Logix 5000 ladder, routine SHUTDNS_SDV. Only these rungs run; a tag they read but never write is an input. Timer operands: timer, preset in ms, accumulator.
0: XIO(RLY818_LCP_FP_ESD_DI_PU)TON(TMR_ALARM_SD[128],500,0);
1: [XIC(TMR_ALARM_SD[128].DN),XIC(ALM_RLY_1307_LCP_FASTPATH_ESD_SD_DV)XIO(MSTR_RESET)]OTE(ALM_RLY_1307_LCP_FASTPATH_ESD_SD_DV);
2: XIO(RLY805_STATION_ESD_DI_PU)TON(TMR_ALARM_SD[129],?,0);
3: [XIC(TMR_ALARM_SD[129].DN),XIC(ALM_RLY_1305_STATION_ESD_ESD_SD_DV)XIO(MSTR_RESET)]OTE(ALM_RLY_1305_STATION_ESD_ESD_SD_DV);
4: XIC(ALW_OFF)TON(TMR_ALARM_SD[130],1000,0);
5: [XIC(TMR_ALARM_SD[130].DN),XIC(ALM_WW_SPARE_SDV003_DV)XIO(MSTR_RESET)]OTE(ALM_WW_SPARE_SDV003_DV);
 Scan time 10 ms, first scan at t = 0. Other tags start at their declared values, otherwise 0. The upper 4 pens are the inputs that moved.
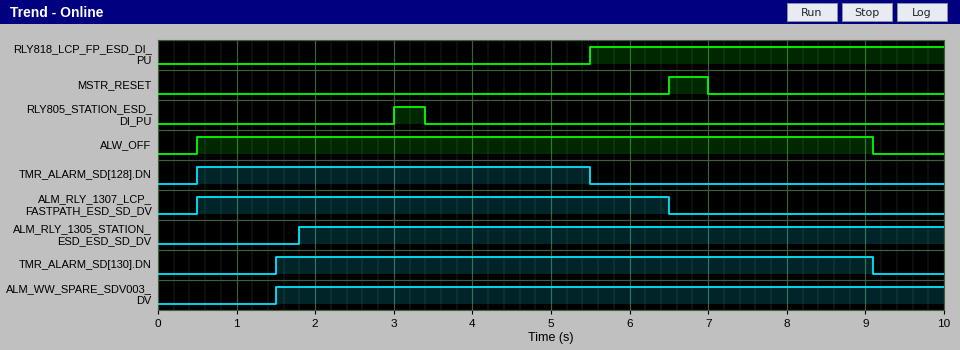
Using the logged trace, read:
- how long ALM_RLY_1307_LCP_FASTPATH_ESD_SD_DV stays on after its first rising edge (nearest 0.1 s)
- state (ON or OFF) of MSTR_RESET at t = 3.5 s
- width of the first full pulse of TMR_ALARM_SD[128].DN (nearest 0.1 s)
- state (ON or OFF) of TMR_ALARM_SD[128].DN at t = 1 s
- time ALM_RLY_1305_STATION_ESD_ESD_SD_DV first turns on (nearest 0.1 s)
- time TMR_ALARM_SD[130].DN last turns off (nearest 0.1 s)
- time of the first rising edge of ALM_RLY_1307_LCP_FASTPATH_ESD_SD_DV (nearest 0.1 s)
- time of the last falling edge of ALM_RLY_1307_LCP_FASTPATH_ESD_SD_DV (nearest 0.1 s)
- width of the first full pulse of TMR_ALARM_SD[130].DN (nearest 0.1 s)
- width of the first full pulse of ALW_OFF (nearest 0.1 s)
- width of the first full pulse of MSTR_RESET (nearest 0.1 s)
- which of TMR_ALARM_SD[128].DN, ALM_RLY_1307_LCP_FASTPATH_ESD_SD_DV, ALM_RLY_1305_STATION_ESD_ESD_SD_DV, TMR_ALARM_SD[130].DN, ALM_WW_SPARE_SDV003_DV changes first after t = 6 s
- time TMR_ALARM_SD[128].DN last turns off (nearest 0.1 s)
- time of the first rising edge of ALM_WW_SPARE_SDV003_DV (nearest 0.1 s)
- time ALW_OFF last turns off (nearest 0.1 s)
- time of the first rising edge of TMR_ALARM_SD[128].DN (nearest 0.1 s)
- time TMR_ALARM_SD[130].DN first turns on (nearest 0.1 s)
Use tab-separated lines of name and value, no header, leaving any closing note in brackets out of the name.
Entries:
how long ALM_RLY_1307_LCP_FASTPATH_ESD_SD_DV stays on after its first rising edge	6.0 s
state (ON or OFF) of MSTR_RESET at t = 3.5 s	OFF
width of the first full pulse of TMR_ALARM_SD[128].DN	5.0 s
state (ON or OFF) of TMR_ALARM_SD[128].DN at t = 1 s	ON
time ALM_RLY_1305_STATION_ESD_ESD_SD_DV first turns on	1.8 s
time TMR_ALARM_SD[130].DN last turns off	9.1 s
time of the first rising edge of ALM_RLY_1307_LCP_FASTPATH_ESD_SD_DV	0.5 s
time of the last falling edge of ALM_RLY_1307_LCP_FASTPATH_ESD_SD_DV	6.5 s
width of the first full pulse of TMR_ALARM_SD[130].DN	7.6 s
width of the first full pulse of ALW_OFF	8.6 s
width of the first full pulse of MSTR_RESET	0.5 s
which of TMR_ALARM_SD[128].DN, ALM_RLY_1307_LCP_FASTPATH_ESD_SD_DV, ALM_RLY_1305_STATION_ESD_ESD_SD_DV, TMR_ALARM_SD[130].DN, ALM_WW_SPARE_SDV003_DV changes first after t = 6 s	ALM_RLY_1307_LCP_FASTPATH_ESD_SD_DV
time TMR_ALARM_SD[128].DN last turns off	5.5 s
time of the first rising edge of ALM_WW_SPARE_SDV003_DV	1.5 s
time ALW_OFF last turns off	9.1 s
time of the first rising edge of TMR_ALARM_SD[128].DN	0.5 s
time TMR_ALARM_SD[130].DN first turns on	1.5 s
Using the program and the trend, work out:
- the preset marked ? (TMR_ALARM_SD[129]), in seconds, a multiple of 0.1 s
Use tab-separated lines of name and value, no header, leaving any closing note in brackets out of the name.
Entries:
the preset marked ? (TMR_ALARM_SD[129]), in seconds, a multiple of 0.1 s	1.8 s
